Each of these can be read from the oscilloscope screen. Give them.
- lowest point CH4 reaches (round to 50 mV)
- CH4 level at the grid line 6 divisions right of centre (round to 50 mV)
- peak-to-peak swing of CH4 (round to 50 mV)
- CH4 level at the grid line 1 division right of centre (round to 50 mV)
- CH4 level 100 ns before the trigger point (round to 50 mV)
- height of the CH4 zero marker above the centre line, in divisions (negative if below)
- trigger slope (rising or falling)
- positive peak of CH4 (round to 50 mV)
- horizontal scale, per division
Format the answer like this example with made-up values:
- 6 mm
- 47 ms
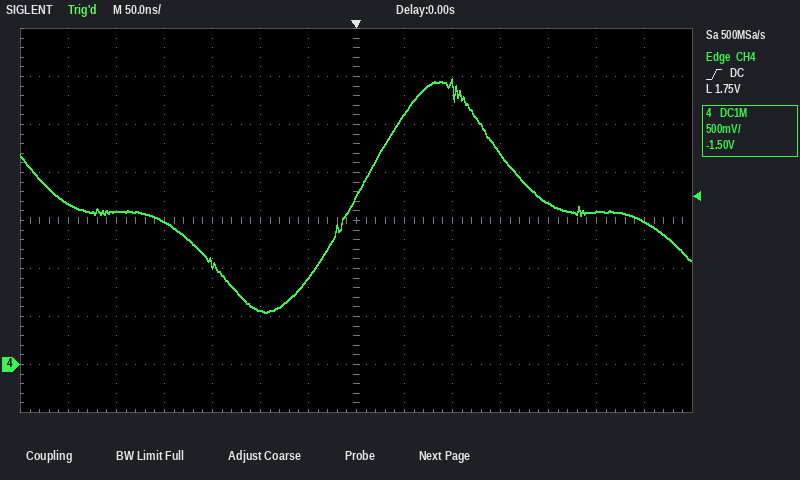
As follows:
- 550 mV
- 1.50 V
- 2.45 V
- 2.60 V
- 550 mV
- -3.0 div
- rising
- 3.00 V
- 50 ns
